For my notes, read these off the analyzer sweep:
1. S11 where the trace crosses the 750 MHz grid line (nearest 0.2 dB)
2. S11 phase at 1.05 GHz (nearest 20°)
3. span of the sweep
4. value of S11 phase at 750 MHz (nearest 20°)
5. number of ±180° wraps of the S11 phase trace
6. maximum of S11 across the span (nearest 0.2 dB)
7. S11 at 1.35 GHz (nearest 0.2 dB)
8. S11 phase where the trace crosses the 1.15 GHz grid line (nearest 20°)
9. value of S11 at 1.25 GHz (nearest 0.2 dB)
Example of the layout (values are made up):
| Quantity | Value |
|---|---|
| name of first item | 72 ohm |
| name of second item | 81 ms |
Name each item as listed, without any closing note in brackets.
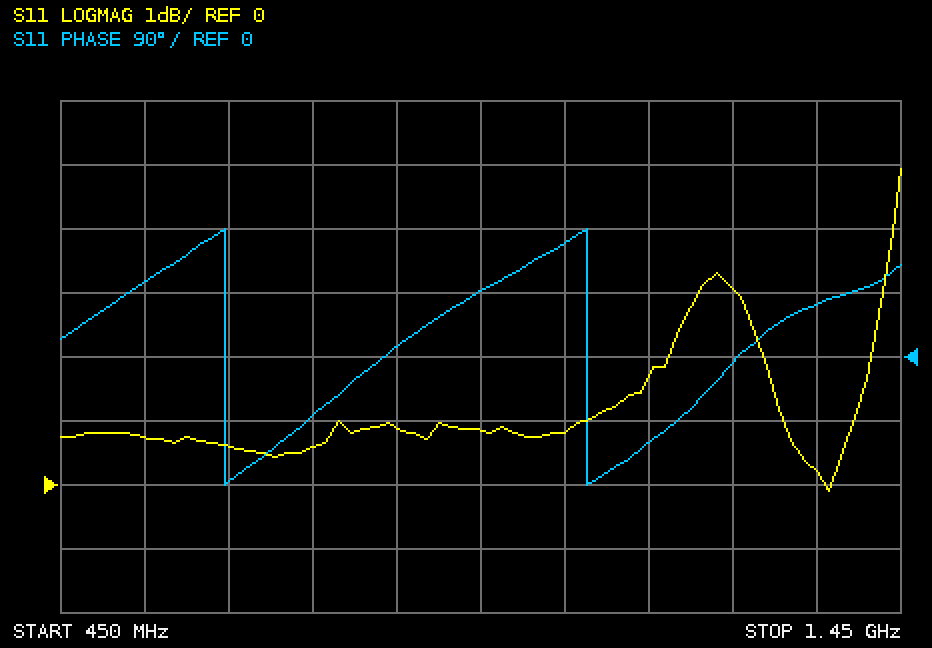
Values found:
| Quantity | Value |
|---|---|
| S11 where the trace crosses the 750 MHz grid line | 0.6 dB |
| S11 phase at 1.05 GHz | 160° |
| span of the sweep | 1 GHz |
| value of S11 phase at 750 MHz | -80° |
| number of ±180° wraps of the S11 phase trace | 2 |
| maximum of S11 across the span | 5.0 dB |
| S11 at 1.35 GHz | 0.2 dB |
| S11 phase where the trace crosses the 1.15 GHz grid line | -120° |
| value of S11 at 1.25 GHz | 3.0 dB |
